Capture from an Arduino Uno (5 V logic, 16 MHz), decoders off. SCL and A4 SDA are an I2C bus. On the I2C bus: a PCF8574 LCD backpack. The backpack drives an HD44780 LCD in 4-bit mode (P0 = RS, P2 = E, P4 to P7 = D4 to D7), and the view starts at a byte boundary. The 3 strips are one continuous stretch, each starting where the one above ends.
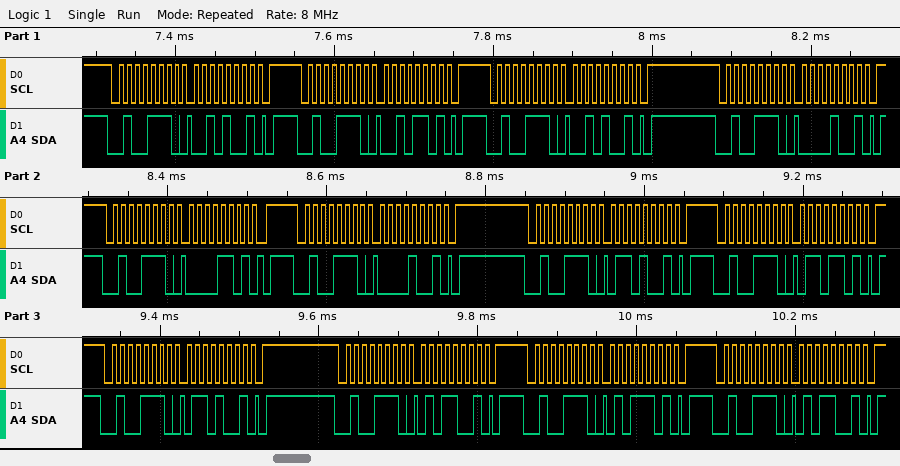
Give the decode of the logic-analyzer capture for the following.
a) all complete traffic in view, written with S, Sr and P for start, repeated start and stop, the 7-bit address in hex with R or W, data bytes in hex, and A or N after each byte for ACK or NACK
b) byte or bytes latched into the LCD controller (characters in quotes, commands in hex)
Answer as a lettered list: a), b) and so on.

a) S 27W A 29 A P S 27W A 2D A P S 27W A 29 A P S 27W A 09 A P S 27W A 0D A P S 27W A 09 A P S 27W A 69 A P S 27W A 6D A P S 27W A 69 A P S 27W A 59 A P S 27W A 5D A P S 27W A 59 A P
b) ' ' 'e'
